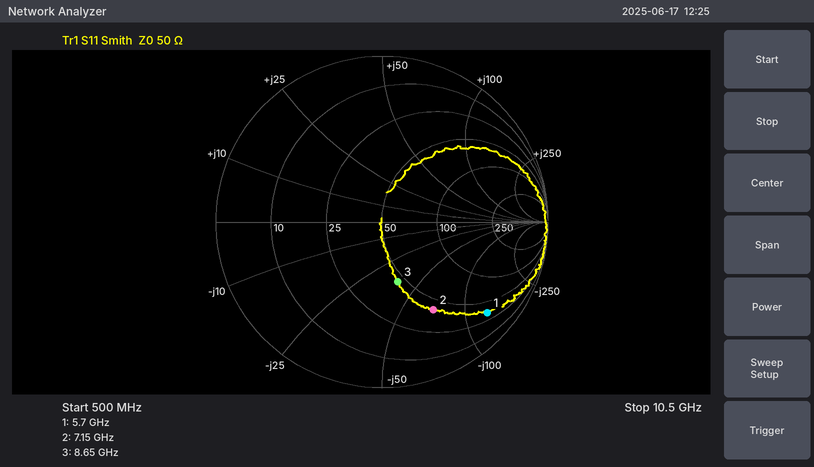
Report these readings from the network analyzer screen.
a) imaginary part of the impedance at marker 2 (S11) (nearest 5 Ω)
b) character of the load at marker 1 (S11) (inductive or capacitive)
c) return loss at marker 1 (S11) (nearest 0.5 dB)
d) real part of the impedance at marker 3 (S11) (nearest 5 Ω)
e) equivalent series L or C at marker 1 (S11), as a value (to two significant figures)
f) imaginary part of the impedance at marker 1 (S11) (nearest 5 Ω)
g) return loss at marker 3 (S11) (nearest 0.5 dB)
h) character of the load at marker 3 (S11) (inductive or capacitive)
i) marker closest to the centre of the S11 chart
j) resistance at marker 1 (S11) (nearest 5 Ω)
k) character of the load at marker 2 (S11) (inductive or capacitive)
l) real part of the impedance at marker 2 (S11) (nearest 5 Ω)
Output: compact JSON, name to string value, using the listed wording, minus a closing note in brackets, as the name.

{"imaginary part of the impedance at marker 2 (S11)": "-70 Ω", "character of the load at marker 1 (S11)": "capacitive", "return loss at marker 1 (S11)": "1.5 dB", "real part of the impedance at marker 3 (S11)": "45 Ω", "equivalent series L or C at marker 1 (S11), as a value": "220 fF", "imaginary part of the impedance at marker 1 (S11)": "-125 Ω", "return loss at marker 3 (S11)": "8.5 dB", "character of the load at marker 3 (S11)": "capacitive", "marker closest to the centre of the S11 chart": "marker 3", "resistance at marker 1 (S11)": "35 Ω", "character of the load at marker 2 (S11)": "capacitive", "real part of the impedance at marker 2 (S11)": "40 Ω"}
